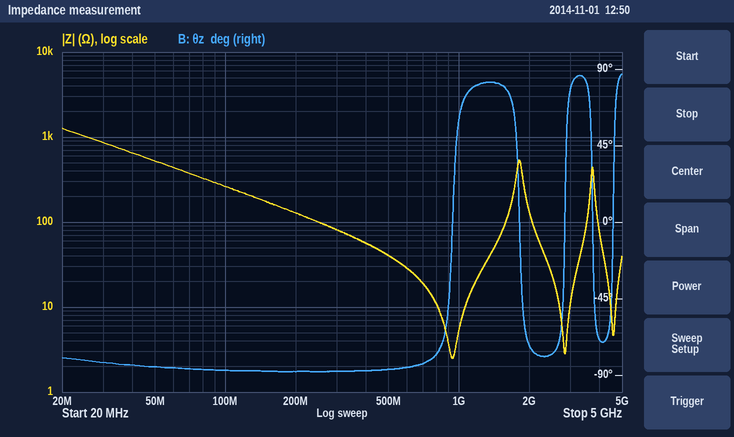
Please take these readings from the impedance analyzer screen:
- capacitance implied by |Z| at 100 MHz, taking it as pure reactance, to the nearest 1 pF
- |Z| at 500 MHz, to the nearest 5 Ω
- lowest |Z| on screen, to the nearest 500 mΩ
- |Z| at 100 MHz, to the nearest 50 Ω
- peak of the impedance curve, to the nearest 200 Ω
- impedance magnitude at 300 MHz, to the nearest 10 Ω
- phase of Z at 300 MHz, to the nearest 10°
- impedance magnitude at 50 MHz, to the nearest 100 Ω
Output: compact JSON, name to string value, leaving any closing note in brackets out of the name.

{"capacitance implied by |Z| at 100 MHz, taking it as pure reactance, to the nearest 1 pF": "6 pF", "|Z| at 500 MHz, to the nearest 5 Ω": "40 Ω", "lowest |Z| on screen, to the nearest 500 mΩ": "2.5 Ω", "|Z| at 100 MHz, to the nearest 50 Ω": "250 Ω", "peak of the impedance curve, to the nearest 200 Ω": "1.2 kΩ", "impedance magnitude at 300 MHz, to the nearest 10 Ω": "80 Ω", "phase of Z at 300 MHz, to the nearest 10°": "-90°", "impedance magnitude at 50 MHz, to the nearest 100 Ω": "500 Ω"}
